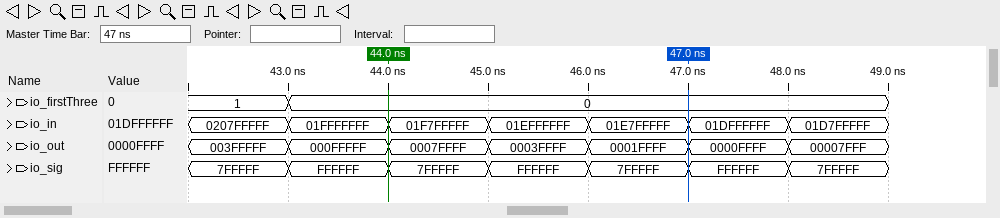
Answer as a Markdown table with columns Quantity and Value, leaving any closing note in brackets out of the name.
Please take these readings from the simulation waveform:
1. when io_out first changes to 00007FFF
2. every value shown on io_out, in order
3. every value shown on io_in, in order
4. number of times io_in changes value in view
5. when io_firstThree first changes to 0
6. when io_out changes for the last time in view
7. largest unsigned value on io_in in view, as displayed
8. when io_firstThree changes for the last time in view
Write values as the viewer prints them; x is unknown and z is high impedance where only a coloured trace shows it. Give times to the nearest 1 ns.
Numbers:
| Quantity | Value |
|---|---|
| when io_out first changes to 00007FFF | 48 ns |
| every value shown on io_out, in order | 003FFFFF, 000FFFFF, 0007FFFF, 0003FFFF, 0001FFFF, 0000FFFF, 00007FFF |
| every value shown on io_in, in order | 0207FFFFF, 01FFFFFFF, 01F7FFFFF, 01EFFFFFF, 01E7FFFFF, 01DFFFFFF, 01D7FFFFF |
| number of times io_in changes value in view | 6 |
| when io_firstThree first changes to 0 | 43 ns |
| when io_out changes for the last time in view | 48 ns |
| largest unsigned value on io_in in view, as displayed | 0207FFFFF |
| when io_firstThree changes for the last time in view | 43 ns |
